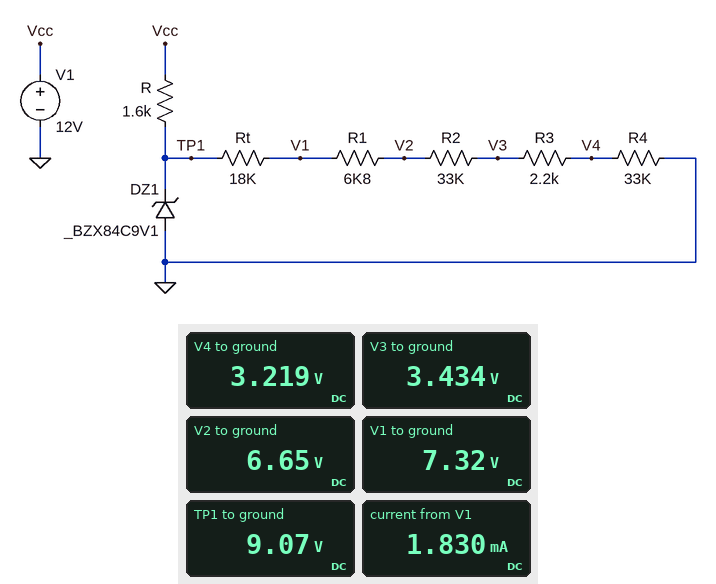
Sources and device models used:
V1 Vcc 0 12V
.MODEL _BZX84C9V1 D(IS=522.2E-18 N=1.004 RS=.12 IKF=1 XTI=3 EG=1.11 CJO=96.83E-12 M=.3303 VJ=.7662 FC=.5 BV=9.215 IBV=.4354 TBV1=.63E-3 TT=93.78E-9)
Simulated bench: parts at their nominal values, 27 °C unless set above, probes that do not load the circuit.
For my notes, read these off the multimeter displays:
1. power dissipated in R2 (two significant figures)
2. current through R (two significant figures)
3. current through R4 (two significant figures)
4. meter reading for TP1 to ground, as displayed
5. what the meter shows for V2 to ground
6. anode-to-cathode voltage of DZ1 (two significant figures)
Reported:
310 µW
1.8 mA
98 µA
9.07 V
6.65 V
-9.1 V
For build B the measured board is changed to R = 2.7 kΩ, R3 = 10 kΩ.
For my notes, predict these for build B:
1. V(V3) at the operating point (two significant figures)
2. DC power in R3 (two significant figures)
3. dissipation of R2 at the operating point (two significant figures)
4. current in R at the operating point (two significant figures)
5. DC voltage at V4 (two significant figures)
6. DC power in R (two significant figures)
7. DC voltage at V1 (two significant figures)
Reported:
3.9 V
81 µW
270 µW
1.1 mA
3.0 V
3.2 mW
7.4 V
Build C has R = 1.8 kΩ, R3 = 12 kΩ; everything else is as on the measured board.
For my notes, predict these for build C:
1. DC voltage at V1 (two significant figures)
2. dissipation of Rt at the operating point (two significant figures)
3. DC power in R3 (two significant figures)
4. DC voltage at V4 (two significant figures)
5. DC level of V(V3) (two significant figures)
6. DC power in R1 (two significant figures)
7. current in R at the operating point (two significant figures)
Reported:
7.5 V
140 µW
93 µW
2.9 V
4.0 V
53 µW
1.6 mA
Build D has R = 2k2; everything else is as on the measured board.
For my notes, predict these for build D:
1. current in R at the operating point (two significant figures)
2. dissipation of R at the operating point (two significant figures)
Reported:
1.3 mA
3.9 mW
